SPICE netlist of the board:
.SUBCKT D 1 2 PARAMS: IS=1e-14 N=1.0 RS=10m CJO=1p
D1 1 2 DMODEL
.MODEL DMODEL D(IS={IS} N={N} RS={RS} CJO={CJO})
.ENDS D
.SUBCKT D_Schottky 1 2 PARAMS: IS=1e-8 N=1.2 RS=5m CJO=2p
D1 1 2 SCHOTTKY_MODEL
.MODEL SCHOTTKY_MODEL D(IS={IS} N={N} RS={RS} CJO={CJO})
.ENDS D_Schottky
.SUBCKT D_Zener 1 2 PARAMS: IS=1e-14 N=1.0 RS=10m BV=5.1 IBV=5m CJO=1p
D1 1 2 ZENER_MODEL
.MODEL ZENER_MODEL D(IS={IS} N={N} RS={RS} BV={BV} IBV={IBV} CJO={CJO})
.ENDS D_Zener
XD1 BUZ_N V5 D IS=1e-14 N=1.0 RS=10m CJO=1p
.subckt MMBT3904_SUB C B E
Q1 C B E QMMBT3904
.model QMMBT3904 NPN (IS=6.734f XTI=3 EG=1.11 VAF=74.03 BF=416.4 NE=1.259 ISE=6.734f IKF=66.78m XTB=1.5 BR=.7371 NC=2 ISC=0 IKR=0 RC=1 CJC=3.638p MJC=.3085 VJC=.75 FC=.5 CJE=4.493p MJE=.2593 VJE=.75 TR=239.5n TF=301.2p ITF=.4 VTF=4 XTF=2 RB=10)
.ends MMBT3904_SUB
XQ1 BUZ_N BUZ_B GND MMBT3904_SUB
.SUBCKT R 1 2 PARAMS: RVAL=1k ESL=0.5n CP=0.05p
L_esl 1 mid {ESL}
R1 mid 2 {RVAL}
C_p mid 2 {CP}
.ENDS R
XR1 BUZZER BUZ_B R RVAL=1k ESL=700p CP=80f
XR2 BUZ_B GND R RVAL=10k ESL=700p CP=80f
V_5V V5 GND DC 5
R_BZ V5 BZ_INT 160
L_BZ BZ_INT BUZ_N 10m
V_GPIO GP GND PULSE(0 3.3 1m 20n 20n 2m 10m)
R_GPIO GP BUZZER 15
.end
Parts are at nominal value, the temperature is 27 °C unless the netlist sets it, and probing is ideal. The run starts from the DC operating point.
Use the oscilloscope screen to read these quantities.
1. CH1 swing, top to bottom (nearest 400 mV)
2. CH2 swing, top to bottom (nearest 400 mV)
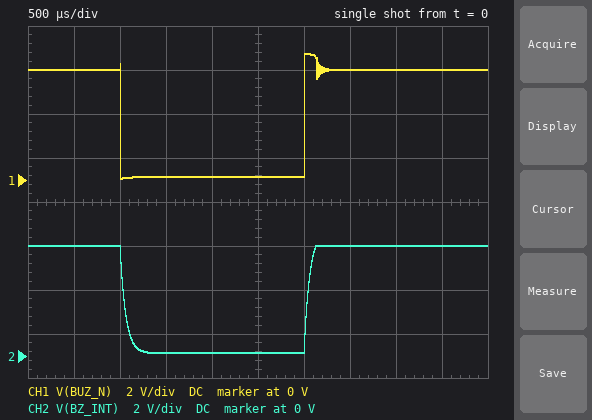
5.6 V
4.8 V
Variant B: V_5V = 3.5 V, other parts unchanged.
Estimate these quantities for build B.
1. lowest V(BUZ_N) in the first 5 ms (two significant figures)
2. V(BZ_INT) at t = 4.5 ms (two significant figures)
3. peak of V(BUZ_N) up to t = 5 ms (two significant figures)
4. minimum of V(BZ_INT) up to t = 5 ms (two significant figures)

25 mV
3.5 V
4.2 V
100 mV
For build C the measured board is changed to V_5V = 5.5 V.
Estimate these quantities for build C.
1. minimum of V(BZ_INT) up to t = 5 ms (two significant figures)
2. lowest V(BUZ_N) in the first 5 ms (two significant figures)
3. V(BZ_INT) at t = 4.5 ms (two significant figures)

130 mV
26 mV
5.5 V
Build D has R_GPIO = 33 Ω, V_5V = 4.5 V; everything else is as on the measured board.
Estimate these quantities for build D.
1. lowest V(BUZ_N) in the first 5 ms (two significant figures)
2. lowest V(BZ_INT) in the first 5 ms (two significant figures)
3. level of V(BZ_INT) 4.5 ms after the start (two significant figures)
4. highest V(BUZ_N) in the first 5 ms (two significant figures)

26 mV
110 mV
4.5 V
5.2 V
